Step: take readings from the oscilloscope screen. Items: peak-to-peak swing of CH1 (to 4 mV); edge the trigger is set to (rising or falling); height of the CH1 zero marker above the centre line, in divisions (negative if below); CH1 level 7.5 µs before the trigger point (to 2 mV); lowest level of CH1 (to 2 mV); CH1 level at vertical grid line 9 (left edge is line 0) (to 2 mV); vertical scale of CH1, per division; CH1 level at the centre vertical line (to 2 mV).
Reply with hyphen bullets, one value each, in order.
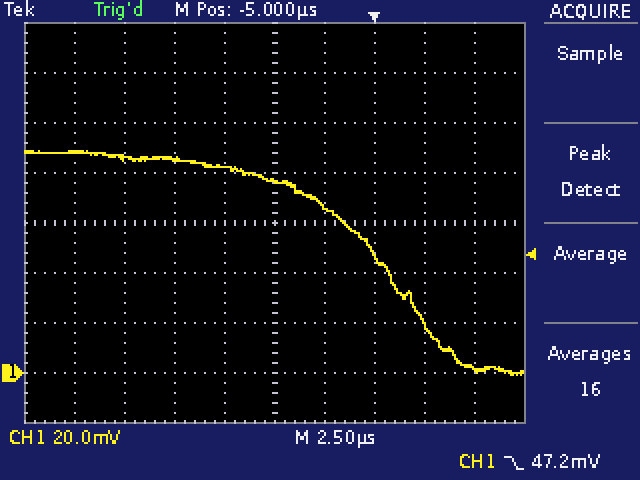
- 88 mV
- falling
- -3.0 div
- 82 mV
- 0 mV
- 2 mV
- 20 mV
- 76 mV
